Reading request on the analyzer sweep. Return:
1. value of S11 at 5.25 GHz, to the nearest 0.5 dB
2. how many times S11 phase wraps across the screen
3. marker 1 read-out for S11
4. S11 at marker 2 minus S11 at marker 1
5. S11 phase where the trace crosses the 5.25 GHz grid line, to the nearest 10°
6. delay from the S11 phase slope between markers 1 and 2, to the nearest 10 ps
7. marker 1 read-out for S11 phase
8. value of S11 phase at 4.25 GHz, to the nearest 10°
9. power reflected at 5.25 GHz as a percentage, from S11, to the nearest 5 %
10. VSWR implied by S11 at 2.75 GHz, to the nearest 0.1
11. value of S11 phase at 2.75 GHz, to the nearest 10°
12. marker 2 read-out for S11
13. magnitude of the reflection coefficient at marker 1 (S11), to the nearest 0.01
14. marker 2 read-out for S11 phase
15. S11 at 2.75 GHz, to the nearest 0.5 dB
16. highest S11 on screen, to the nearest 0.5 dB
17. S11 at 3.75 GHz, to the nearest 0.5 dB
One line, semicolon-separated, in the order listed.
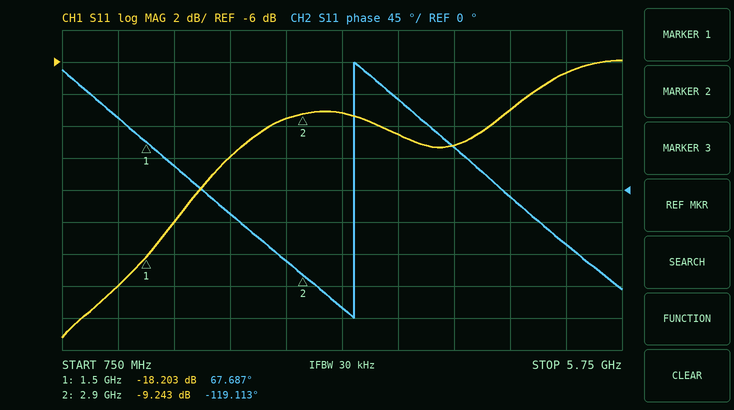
-6.5 dB; 1; -18.203 dB; 8.960 dB; -80°; 370 ps; 67.687°; 60°; 20 %; 2.0; -100°; -9.243 dB; 0.12; -119.113°; -9.5 dB; -6.0 dB; -10.5 dB
